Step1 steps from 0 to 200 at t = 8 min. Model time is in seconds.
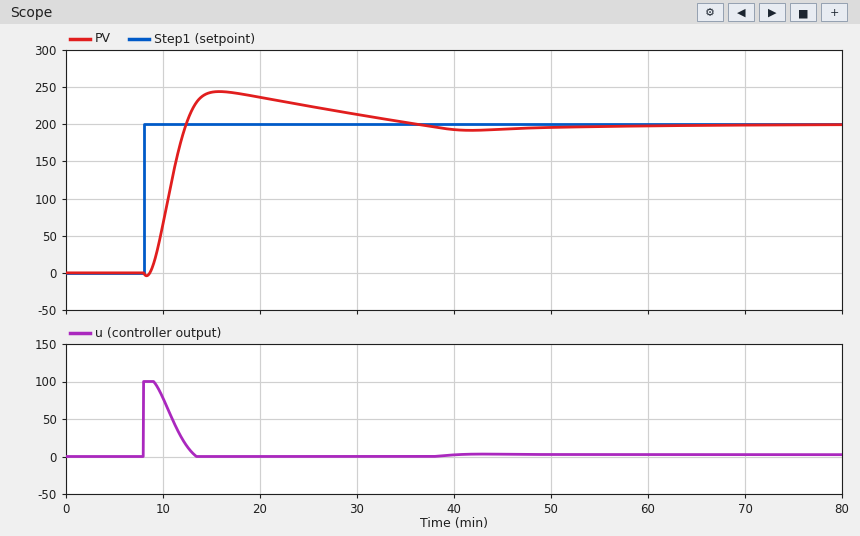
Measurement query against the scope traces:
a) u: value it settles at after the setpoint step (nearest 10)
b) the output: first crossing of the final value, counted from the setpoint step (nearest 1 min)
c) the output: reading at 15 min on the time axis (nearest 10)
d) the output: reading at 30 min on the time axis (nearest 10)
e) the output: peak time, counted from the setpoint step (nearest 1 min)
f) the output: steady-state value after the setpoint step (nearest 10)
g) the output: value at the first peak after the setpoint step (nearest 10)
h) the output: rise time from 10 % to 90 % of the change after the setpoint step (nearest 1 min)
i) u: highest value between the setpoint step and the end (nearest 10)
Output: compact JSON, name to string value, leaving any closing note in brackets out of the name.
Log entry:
{"u: value it settles at after the setpoint step": "0", "the output: first crossing of the final value, counted from the setpoint step": "4 min", "the output: reading at 15 min on the time axis": "240", "the output: reading at 30 min on the time axis": "210", "the output: peak time, counted from the setpoint step": "8 min", "the output: steady-state value after the setpoint step": "200", "the output: value at the first peak after the setpoint step": "240", "the output: rise time from 10 % to 90 % of the change after the setpoint step": "3 min", "u: highest value between the setpoint step and the end": "100"}
